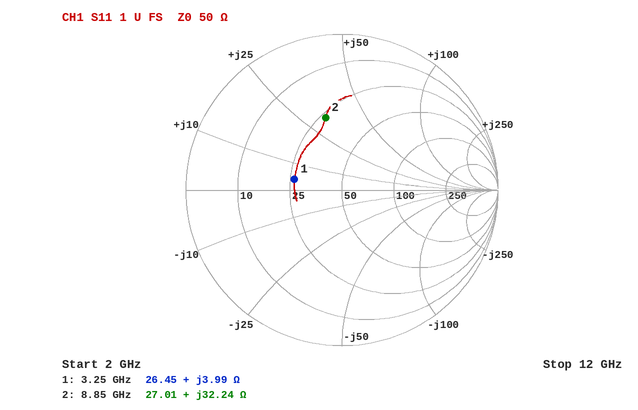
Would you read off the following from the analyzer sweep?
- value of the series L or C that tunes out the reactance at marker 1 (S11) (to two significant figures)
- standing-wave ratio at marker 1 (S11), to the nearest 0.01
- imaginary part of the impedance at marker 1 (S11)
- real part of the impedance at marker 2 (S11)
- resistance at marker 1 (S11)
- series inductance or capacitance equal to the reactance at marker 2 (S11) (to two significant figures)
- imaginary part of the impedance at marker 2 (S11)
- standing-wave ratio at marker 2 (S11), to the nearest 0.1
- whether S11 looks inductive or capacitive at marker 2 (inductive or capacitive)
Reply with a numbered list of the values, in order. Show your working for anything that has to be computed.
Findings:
1. C = 1/(2π × 3.25 GHz × 3.99 Ω) ≈ 12 pF
2. 1.91
3. +3.99 Ω
4. 27.01 Ω
5. 26.45 Ω
6. L = 32.24 Ω/(2π × 8.85 GHz) ≈ 580 pH
7. +32.24 Ω
8. 2.8
9. inductive
